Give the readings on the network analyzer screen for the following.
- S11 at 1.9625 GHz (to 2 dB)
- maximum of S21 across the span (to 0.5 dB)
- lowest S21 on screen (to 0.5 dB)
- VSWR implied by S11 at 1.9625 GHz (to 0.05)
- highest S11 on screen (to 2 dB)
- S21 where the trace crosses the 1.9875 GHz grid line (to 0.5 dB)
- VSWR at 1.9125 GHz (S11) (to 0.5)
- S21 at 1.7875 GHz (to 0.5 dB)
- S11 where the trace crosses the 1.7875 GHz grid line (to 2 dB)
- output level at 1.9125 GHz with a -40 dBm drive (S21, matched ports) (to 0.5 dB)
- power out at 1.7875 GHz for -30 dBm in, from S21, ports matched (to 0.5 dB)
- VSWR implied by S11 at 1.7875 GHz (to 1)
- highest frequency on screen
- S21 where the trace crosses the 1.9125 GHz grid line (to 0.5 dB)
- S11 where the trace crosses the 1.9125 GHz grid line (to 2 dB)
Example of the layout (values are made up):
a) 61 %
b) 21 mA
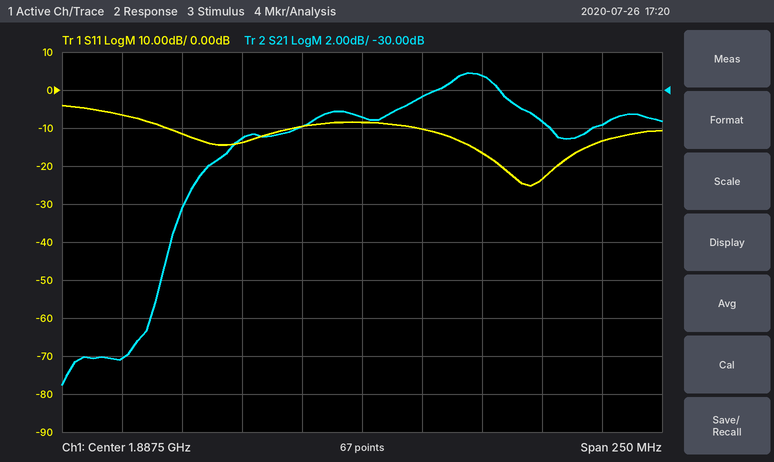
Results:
a) -24 dB
b) -29.0 dB
c) -45.5 dB
d) 1.15
e) -4 dB
f) -32.0 dB
g) 2.0
h) -44.0 dB
i) -6 dB
j) -70.5 dBm
k) -74.0 dBm
l) 3
m) 2.0125 GHz
n) -30.5 dB
o) -10 dB
